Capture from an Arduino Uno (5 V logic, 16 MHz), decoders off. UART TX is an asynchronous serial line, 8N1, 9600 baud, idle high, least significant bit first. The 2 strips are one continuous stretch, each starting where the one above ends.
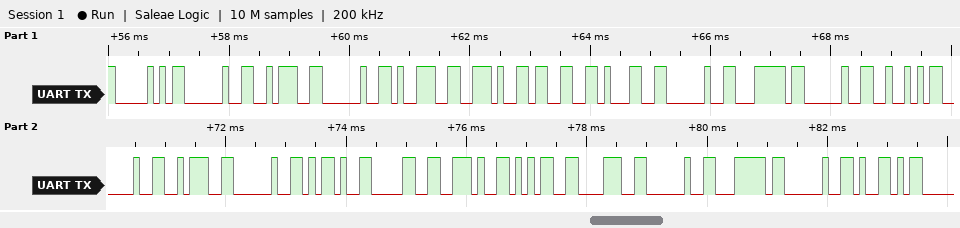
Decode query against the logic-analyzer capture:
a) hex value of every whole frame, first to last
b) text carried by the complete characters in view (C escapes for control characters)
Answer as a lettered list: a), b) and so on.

a) 50 20 3A 20 39 2E 33 31 20 7C 20 52 20 3A 20 2D 30 2E 35 38 20 7C 20 59
b) "P : 9.31 | R : -0.58 | Y"
